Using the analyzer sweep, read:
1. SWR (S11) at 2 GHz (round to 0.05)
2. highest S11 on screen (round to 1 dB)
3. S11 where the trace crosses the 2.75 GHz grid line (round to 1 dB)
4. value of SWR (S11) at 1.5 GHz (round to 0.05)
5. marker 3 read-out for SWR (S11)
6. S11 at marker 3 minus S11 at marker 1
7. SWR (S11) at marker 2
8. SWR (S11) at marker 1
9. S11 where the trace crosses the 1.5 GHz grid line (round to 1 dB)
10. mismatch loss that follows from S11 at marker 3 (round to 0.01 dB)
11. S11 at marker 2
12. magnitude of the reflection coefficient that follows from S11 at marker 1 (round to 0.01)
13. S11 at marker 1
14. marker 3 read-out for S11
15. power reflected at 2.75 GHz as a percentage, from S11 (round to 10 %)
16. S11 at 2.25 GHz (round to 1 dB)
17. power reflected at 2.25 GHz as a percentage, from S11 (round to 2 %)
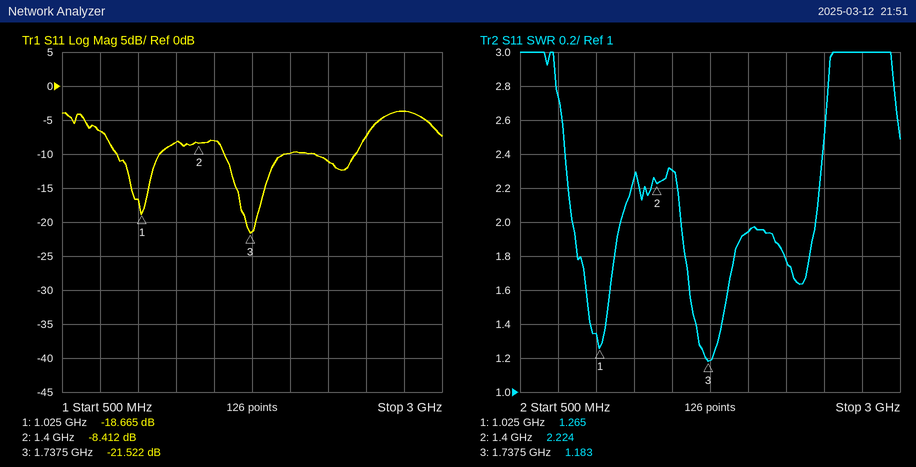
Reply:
1.95
-4 dB
-4 dB
2.30
1.183
-2.857 dB
2.224
1.265
-8 dB
0.03 dB
-8.412 dB
0.12
-18.665 dB
-21.522 dB
40 %
-11 dB
8 %
